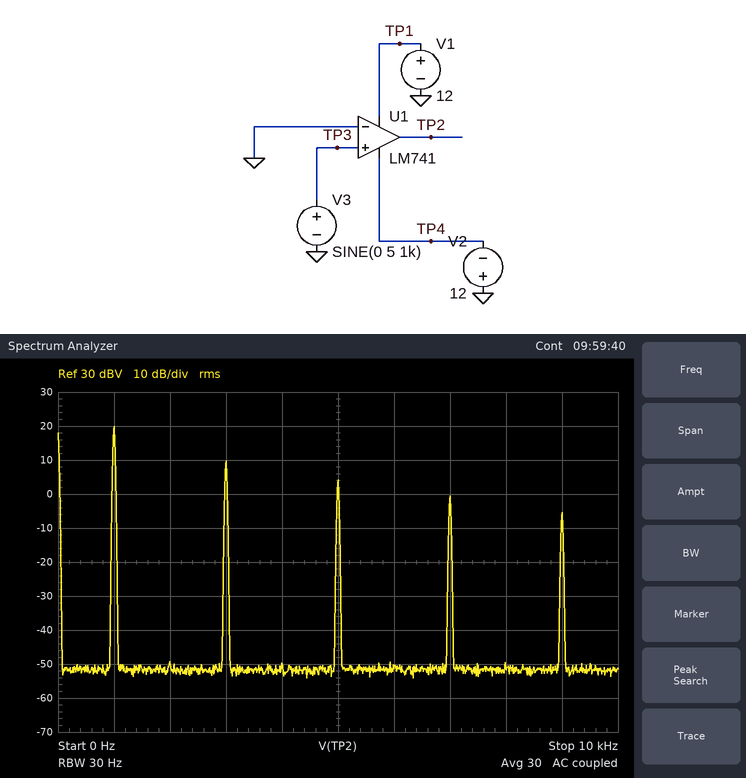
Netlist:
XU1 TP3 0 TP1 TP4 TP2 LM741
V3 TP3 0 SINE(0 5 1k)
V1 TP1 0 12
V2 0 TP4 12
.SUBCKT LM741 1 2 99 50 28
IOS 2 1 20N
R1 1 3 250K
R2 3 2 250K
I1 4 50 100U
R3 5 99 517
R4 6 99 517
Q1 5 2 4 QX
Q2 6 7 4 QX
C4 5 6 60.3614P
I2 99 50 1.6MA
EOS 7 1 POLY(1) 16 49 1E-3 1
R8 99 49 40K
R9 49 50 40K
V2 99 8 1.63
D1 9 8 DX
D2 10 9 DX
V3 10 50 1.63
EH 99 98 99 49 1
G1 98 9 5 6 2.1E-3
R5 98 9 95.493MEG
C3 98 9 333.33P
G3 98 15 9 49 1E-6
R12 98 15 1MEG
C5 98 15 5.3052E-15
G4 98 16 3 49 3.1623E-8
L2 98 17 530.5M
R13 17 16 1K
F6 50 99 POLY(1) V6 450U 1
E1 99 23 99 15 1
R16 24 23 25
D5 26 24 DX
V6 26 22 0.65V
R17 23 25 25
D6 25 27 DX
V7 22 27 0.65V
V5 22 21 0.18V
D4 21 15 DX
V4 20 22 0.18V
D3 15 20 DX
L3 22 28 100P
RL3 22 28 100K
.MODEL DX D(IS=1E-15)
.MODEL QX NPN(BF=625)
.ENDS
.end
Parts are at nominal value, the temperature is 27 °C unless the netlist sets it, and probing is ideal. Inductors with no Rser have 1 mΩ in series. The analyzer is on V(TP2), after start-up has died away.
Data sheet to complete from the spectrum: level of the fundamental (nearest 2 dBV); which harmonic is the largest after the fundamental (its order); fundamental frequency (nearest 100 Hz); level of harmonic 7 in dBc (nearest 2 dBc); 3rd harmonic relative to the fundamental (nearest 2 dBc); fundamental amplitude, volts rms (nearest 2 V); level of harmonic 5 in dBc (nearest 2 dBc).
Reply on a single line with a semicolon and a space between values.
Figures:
20 dBV; 3; 1.0 kHz; -20 dBc; -10 dBc; 10 V; -16 dBc
